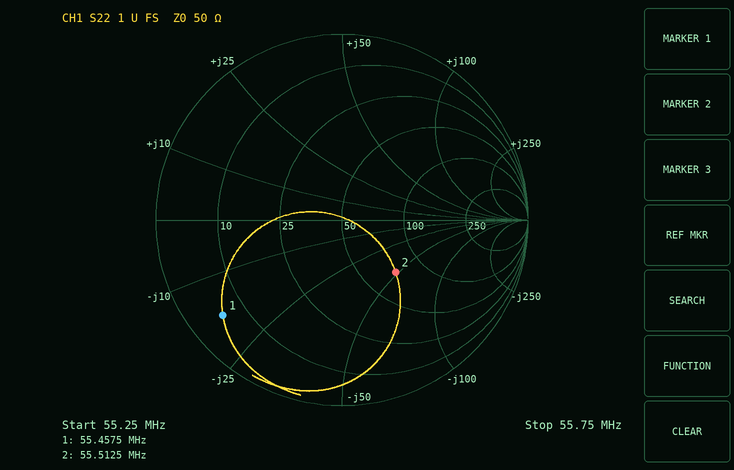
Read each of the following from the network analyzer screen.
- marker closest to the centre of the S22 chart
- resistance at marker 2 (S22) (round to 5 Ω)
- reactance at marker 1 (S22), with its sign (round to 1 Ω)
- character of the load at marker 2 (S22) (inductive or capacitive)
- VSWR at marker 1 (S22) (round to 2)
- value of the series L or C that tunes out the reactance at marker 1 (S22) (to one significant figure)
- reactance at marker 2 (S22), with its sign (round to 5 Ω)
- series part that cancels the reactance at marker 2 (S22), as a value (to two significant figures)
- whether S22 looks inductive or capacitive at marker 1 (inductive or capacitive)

marker 2
70 Ω
-17 Ω
capacitive
10
50 nH
-50 Ω
140 nH
capacitive
